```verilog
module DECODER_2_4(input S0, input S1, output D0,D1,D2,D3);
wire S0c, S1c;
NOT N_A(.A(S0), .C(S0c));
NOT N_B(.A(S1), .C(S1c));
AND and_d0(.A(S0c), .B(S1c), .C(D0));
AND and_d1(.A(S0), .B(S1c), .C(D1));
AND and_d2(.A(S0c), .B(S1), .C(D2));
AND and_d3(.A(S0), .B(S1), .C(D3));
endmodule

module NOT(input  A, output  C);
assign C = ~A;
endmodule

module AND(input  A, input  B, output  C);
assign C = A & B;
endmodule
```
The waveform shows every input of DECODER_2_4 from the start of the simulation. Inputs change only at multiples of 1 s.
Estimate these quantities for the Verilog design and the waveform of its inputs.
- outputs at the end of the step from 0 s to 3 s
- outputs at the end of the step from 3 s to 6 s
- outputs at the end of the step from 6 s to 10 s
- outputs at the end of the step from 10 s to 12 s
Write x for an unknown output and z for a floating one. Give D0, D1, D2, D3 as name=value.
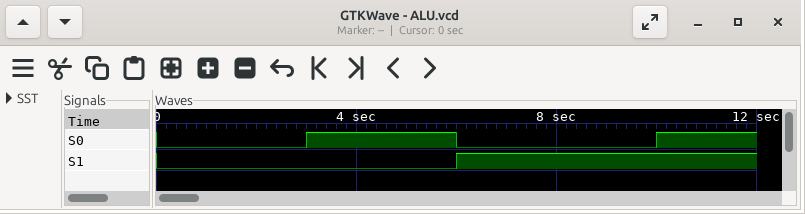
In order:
D0=1, D1=0, D2=0, D3=0
D0=0, D1=1, D2=0, D3=0
D0=0, D1=0, D2=1, D3=0
D0=0, D1=0, D2=0, D3=1
